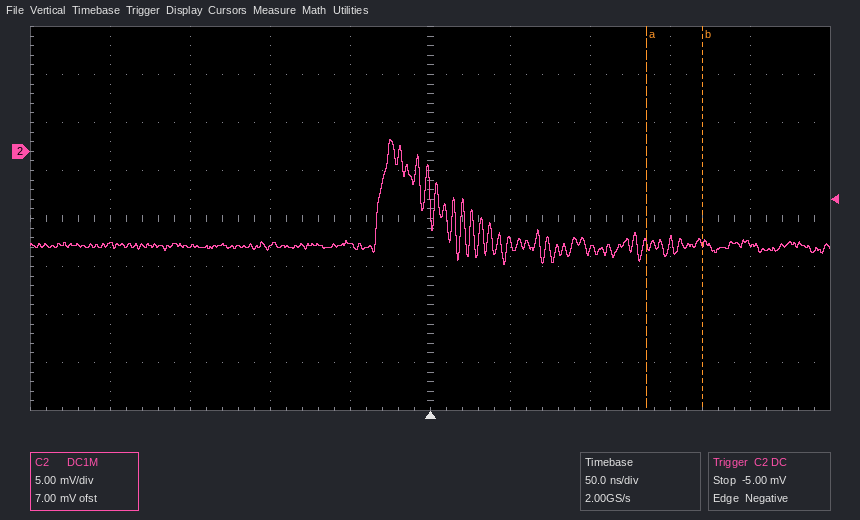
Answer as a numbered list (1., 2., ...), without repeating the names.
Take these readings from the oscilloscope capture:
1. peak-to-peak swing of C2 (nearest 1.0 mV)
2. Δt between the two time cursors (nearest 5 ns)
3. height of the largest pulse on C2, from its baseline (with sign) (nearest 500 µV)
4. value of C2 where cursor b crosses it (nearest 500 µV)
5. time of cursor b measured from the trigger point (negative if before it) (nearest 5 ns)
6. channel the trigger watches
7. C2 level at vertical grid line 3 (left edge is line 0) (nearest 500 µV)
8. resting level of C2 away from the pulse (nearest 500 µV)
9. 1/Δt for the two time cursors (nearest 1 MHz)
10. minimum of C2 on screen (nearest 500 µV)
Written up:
1. 13.0 mV
2. 35 ns
3. +11.0 mV
4. -9.5 mV
5. +170 ns
6. C2
7. -10.0 mV
8. -10.0 mV
9. 29 MHz
10. -12.0 mV
